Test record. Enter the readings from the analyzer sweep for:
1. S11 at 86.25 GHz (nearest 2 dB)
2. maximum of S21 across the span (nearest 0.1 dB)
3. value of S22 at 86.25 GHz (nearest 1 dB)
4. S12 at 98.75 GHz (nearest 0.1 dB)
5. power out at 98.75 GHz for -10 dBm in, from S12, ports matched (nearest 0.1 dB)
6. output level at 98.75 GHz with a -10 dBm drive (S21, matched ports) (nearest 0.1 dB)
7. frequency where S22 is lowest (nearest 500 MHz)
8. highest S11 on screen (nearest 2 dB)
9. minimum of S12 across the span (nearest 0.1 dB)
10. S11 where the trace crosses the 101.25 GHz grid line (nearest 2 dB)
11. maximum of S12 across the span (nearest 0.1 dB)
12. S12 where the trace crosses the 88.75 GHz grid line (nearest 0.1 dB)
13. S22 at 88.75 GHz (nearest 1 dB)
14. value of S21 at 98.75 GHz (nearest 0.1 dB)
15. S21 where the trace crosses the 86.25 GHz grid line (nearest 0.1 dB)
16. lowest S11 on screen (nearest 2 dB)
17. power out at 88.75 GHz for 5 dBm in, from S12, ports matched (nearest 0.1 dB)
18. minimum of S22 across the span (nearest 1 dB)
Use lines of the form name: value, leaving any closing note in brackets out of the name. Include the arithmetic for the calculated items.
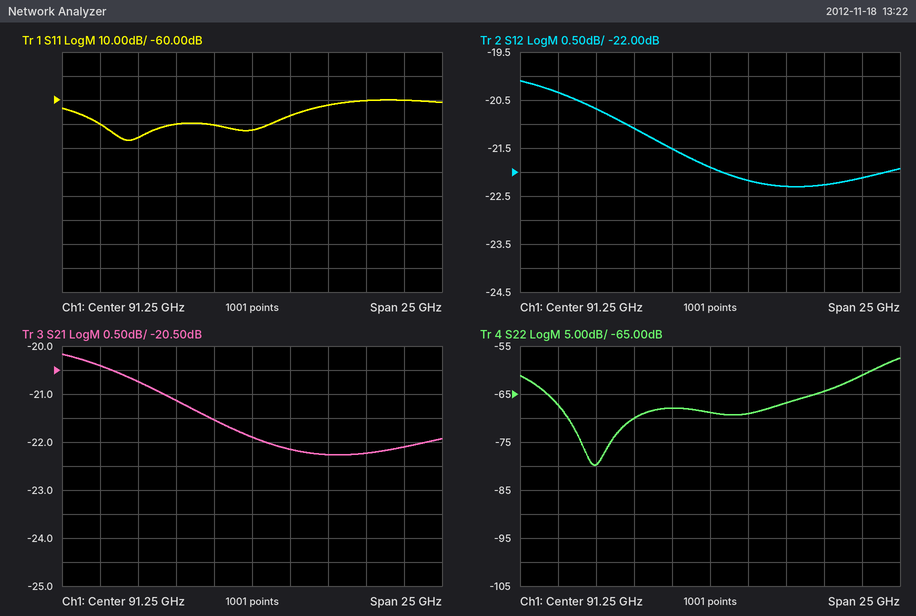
S11 at 86.25 GHz: -70 dB
maximum of S21 across the span: -20.2 dB
value of S22 at 86.25 GHz: -70 dB
S12 at 98.75 GHz: -22.3 dB
power out at 98.75 GHz for -10 dBm in, from S12, ports matched: -10 dBm + (-22.3 dB) = -32.3 dBm
output level at 98.75 GHz with a -10 dBm drive (S21, matched ports): -10 dBm + (-22.2 dB) = -32.2 dBm
frequency where S22 is lowest: 83.5 GHz
highest S11 on screen: -60 dB
minimum of S12 across the span: -22.3 dB
S11 where the trace crosses the 101.25 GHz grid line: -60 dB
maximum of S12 across the span: -20.1 dB
S12 where the trace crosses the 88.75 GHz grid line: -21.5 dB
S22 at 88.75 GHz: -68 dB
value of S21 at 98.75 GHz: -22.2 dB
S21 where the trace crosses the 86.25 GHz grid line: -21.1 dB
lowest S11 on screen: -76 dB
power out at 88.75 GHz for 5 dBm in, from S12, ports matched: 5 dBm + (-21.5 dB) = -16.5 dBm
minimum of S22 across the span: -80 dB
